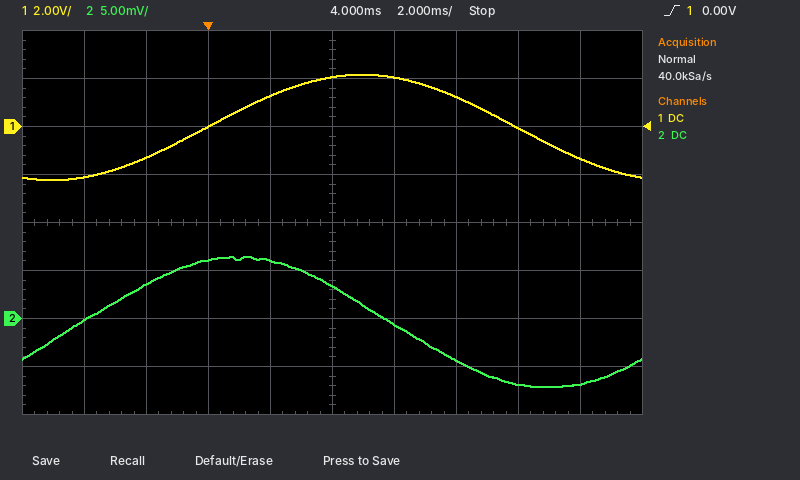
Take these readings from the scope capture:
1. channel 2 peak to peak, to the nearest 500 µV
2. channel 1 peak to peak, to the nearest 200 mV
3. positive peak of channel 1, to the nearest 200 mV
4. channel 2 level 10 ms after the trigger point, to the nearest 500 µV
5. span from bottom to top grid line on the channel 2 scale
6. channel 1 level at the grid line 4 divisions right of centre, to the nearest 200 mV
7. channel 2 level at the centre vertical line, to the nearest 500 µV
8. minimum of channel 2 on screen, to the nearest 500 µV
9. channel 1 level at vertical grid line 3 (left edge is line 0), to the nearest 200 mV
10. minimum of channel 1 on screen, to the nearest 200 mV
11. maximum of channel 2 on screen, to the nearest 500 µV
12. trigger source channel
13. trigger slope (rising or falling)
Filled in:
13.5 mV
4.4 V
2.2 V
-7.0 mV
40 mV
-1.4 V
3.5 mV
-7.0 mV
0.0 V
-2.2 V
6.5 mV
channel 1
rising
